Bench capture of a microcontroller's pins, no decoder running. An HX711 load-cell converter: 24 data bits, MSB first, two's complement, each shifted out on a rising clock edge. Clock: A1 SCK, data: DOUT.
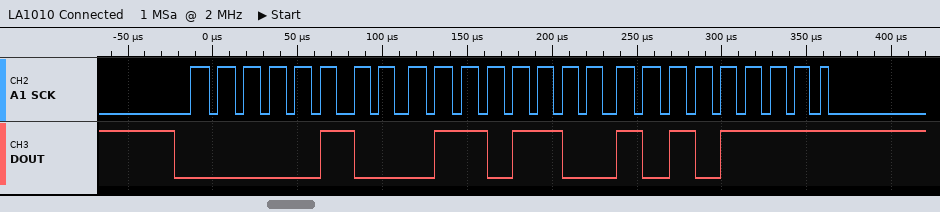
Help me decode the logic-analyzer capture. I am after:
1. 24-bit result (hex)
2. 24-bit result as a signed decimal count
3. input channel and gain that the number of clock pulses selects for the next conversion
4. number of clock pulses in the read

0x046CAF
289967
channel A, gain 128
25
